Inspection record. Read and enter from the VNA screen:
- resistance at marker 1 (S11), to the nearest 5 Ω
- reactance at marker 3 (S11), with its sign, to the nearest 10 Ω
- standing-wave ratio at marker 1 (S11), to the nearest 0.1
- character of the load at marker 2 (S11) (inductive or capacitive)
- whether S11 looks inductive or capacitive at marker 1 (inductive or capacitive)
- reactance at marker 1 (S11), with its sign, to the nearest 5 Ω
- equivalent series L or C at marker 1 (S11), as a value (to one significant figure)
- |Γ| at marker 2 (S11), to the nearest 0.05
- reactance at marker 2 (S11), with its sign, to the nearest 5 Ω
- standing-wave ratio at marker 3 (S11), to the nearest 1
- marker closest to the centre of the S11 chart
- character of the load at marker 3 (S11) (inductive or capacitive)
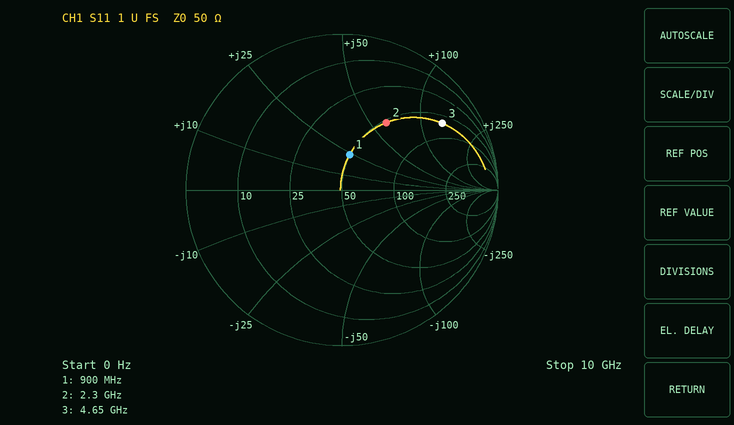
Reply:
50 Ω
+140 Ω
1.6
inductive
inductive
+25 Ω
4 nH
0.50
+60 Ω
8
marker 1
inductive
